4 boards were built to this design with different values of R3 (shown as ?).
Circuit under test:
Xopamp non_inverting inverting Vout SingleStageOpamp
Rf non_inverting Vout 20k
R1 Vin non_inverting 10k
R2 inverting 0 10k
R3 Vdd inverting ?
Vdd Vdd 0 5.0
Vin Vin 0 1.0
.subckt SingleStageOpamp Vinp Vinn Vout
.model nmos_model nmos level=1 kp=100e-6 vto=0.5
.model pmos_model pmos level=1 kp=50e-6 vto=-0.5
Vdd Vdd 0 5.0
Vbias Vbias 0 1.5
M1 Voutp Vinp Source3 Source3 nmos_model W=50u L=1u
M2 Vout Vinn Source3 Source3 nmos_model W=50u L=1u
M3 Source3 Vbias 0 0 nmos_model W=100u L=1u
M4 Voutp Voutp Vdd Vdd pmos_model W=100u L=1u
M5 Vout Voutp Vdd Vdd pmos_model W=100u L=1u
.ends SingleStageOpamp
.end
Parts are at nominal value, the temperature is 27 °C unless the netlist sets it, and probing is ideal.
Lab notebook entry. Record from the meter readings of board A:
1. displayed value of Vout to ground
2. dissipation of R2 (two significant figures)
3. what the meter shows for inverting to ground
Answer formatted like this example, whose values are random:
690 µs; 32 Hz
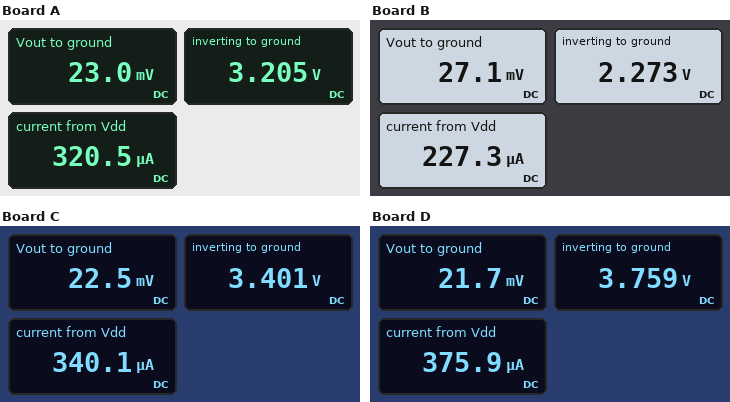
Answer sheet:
23.0 mV; 1.0 mW; 3.205 V
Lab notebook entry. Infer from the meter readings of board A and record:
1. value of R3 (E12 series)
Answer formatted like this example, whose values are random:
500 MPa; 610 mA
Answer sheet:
5.6 kΩ
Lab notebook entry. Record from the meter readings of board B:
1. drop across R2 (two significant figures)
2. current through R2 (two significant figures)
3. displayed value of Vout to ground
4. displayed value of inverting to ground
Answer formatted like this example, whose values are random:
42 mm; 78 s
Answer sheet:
2.3 V; 230 µA; 27.1 mV; 2.273 V
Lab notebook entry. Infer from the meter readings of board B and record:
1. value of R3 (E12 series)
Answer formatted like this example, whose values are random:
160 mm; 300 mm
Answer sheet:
12 kΩ
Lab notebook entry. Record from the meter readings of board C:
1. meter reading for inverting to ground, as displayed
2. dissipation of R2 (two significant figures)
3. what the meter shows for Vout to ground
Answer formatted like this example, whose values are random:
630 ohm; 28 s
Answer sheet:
3.401 V; 1.2 mW; 22.5 mV
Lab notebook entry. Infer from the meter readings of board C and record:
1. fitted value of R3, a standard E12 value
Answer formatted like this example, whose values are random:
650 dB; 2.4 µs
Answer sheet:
4.7 kΩ
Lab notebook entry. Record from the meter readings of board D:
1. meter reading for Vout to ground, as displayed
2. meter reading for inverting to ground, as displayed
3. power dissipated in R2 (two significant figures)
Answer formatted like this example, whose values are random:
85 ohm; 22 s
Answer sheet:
21.7 mV; 3.759 V; 1.4 mW
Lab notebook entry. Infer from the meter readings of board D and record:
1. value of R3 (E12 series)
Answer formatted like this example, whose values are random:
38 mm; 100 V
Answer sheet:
3.3 kΩ
